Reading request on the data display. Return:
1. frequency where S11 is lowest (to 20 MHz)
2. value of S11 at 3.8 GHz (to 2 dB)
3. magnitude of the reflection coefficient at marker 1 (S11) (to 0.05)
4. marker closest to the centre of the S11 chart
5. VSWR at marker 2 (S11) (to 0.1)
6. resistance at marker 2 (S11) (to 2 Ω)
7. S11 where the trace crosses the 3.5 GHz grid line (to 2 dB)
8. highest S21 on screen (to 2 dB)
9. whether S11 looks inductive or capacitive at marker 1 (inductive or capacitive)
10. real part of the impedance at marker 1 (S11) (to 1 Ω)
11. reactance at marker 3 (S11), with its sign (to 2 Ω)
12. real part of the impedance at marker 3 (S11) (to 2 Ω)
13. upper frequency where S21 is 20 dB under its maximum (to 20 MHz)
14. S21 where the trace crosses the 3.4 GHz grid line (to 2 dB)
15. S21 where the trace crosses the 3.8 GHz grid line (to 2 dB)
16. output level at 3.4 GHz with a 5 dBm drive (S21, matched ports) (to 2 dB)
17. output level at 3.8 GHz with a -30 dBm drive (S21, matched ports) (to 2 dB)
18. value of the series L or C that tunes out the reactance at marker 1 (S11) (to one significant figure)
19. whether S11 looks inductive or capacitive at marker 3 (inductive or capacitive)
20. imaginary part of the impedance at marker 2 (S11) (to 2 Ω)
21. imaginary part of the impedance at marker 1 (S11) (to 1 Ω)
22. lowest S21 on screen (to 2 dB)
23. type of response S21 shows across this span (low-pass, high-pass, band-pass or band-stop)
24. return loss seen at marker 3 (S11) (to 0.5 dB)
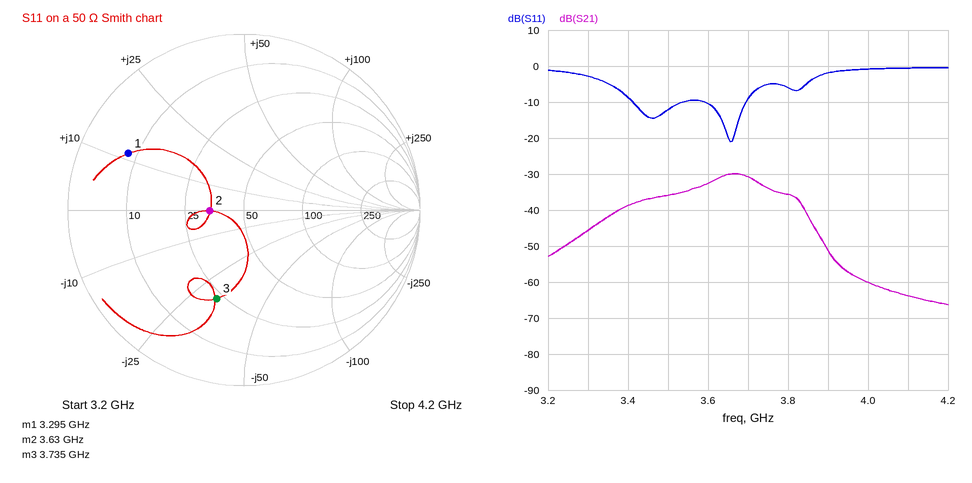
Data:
3.66 GHz
-6 dB
0.75
marker 2
1.5
34 Ω
-12 dB
-30 dB
inductive
8 Ω
-32 Ω
22 Ω
3.90 GHz
-38 dB
-36 dB
-34 dBm
-66 dBm
4 pF
capacitive
0 Ω
+11 Ω
-66 dB
band-pass
5.5 dB
